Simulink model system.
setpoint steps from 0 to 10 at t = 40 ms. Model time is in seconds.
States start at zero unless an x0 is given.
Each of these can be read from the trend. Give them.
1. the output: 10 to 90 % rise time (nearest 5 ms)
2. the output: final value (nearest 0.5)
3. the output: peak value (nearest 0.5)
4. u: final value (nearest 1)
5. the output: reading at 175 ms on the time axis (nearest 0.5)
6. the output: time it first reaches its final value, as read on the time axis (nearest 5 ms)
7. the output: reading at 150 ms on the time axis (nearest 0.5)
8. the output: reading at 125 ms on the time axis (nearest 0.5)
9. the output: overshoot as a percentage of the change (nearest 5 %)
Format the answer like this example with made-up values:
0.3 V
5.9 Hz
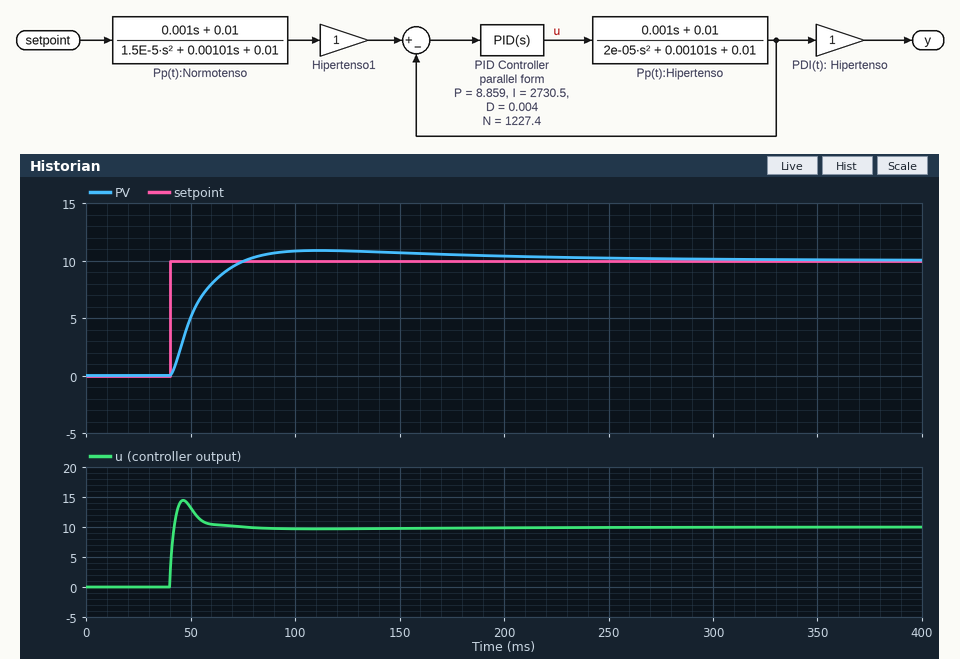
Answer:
25 ms
10.0
11.0
10
10.5
75 ms
10.5
11.0
10 %
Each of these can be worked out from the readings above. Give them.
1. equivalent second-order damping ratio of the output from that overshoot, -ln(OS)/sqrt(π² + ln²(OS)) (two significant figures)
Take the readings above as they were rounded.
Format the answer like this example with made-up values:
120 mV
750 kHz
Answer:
0.59
